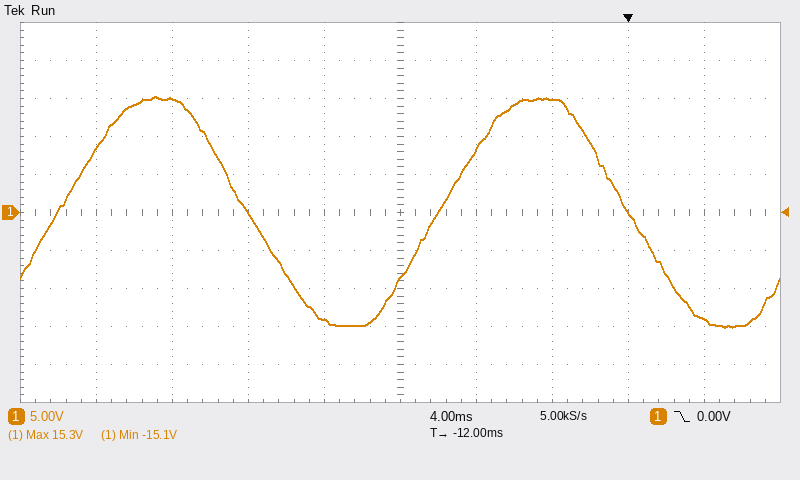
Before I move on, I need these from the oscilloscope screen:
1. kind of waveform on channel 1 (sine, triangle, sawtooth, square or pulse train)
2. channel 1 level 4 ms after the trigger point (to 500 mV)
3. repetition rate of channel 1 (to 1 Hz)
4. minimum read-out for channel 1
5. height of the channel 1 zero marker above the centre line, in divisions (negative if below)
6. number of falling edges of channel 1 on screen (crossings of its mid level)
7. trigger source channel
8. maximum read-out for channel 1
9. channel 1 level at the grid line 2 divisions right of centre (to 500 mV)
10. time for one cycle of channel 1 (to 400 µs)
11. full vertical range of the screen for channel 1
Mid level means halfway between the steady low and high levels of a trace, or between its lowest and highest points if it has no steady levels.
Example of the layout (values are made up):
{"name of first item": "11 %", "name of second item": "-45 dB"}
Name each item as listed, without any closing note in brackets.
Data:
{"kind of waveform on channel 1": "sine", "channel 1 level 4 ms after the trigger point": "-14.0 V", "repetition rate of channel 1": "50 Hz", "minimum read-out for channel 1": "-15.1 V", "height of the channel 1 zero marker above the centre line, in divisions": "0.0 div", "number of falling edges of channel 1 on screen": "2", "trigger source channel": "channel 1", "maximum read-out for channel 1": "15.3 V", "channel 1 level at the grid line 2 divisions right of centre": "15.0 V", "time for one cycle of channel 1": "20.0 ms", "full vertical range of the screen for channel 1": "50 V"}
